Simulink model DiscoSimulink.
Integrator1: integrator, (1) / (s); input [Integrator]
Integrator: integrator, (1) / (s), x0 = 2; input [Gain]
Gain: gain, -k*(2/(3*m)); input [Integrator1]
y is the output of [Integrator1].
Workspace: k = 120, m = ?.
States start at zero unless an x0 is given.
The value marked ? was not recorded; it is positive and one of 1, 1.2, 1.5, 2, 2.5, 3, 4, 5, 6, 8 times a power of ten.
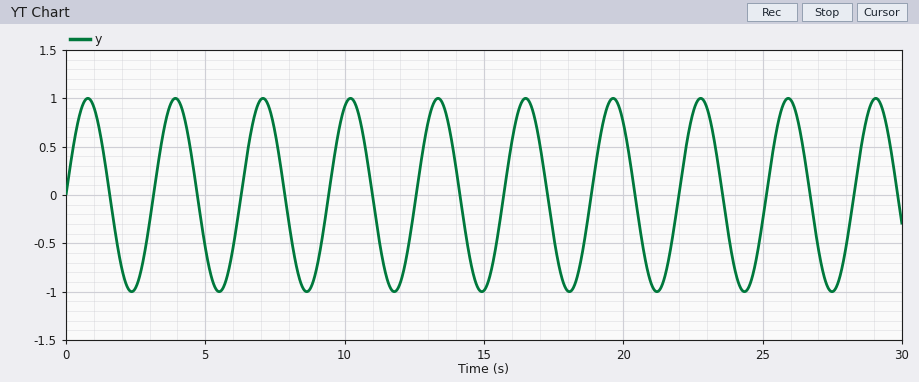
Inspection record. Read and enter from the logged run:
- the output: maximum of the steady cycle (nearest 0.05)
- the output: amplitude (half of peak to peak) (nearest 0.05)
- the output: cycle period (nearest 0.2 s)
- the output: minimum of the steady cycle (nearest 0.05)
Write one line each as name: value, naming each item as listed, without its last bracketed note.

the output: maximum of the steady cycle: 1.00
the output: amplitude (half of peak to peak): 1.00
the output: cycle period: 3.2 s
the output: minimum of the steady cycle: -1.00
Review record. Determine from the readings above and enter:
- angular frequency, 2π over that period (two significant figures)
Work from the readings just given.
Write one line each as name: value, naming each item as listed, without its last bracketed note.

angular frequency, 2π over that period: 2.0 rad/s
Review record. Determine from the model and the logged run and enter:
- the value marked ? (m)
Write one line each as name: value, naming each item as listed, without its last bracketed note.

the value marked ?: 20
